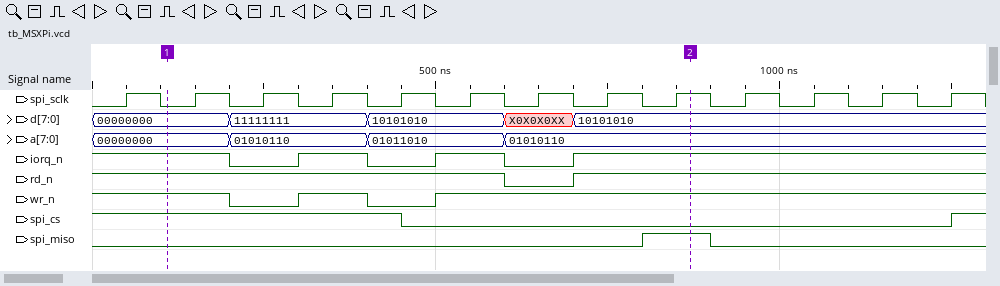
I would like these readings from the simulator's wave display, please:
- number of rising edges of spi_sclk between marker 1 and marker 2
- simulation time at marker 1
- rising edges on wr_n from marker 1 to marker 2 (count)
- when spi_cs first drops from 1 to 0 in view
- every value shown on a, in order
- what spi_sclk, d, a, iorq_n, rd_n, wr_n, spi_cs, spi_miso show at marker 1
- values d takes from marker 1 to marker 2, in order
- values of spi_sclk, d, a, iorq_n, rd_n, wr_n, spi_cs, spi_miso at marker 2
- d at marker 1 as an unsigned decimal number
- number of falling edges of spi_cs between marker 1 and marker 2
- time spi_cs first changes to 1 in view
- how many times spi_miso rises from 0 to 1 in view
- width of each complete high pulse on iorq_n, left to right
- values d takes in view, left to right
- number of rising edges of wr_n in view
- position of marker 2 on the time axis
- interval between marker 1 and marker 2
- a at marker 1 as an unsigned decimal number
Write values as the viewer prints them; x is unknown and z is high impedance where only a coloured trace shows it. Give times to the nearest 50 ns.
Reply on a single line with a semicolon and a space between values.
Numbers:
8; 100 ns; 2; 450 ns; 00000000, 01010110, 01011010, 01010110; spi_sclk=0, d=00000000, a=00000000, iorq_n=1, rd_n=1, wr_n=1, spi_cs=1, spi_miso=0; 00000000, 11111111, 10101010, X0X0X0XX, 10101010; spi_sclk=1, d=10101010, a=01010110, iorq_n=1, rd_n=1, wr_n=1, spi_cs=0, spi_miso=1; 0; 1; 1250 ns; 1; 100 ns, 100 ns; 00000000, 11111111, 10101010, X0X0X0XX, 10101010; 2; 850 ns; 750 ns; 0
